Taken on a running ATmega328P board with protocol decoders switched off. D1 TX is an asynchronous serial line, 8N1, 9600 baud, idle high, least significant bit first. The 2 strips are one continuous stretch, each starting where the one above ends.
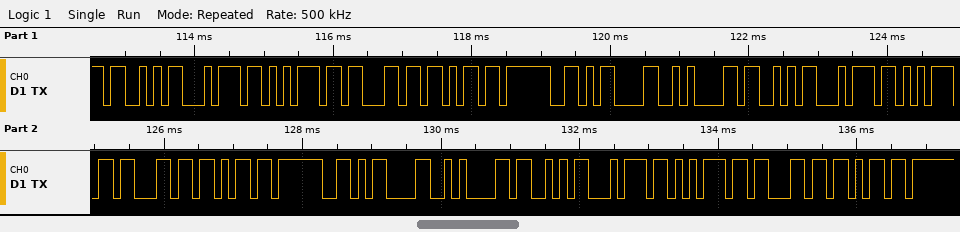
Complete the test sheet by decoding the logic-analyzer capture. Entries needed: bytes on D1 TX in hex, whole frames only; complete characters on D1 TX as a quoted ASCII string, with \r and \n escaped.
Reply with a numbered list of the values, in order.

1. 0x53 0x74 0x75 0x63 0x6B 0x3F 0x0D 0x0A 0x53 0x74 0x75 0x63 0x6B 0x3F 0x0D 0x0A 0x53 0x74 0x75 0x63 0x6B
2. "Stuck?\r\nStuck?\r\nStuck"
